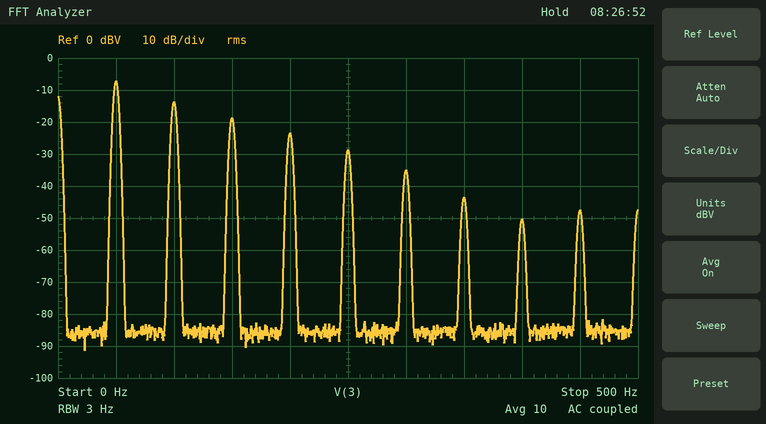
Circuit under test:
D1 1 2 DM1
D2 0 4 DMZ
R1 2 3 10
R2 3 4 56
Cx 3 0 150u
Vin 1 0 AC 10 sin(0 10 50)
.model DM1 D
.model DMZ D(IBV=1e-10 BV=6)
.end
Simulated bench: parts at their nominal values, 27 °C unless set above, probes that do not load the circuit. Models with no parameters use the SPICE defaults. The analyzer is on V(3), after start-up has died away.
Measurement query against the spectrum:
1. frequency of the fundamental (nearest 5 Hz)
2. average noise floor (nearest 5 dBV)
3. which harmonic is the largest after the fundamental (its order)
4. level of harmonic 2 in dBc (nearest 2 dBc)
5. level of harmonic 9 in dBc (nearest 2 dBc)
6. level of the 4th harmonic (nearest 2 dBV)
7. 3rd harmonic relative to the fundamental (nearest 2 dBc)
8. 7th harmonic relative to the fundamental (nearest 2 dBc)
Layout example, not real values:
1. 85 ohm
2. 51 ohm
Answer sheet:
1. 50 Hz
2. -85 dBV
3. 2
4. -6 dBc
5. -40 dBc
6. -24 dBV
7. -12 dBc
8. -36 dBc
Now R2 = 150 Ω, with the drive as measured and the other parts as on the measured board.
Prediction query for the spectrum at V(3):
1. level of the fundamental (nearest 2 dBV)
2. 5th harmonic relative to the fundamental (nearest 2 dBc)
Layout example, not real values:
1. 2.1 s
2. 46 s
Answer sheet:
1. -10 dBV
2. -20 dBc
